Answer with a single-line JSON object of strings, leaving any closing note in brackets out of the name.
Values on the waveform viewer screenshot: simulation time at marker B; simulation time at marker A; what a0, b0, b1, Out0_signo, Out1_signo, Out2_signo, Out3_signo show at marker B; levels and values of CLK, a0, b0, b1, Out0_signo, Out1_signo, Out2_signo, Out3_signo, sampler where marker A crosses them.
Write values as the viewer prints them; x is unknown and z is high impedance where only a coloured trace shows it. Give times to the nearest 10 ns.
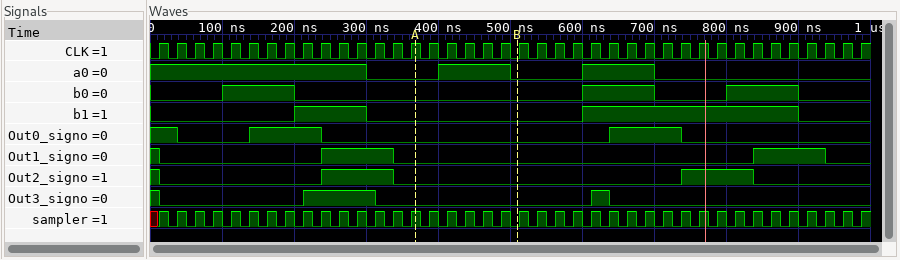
{"simulation time at marker B": "510 ns", "simulation time at marker A": "370 ns", "what a0, b0, b1, Out0_signo, Out1_signo, Out2_signo, Out3_signo show at marker B": "a0=0, b0=0, b1=0, Out0_signo=0, Out1_signo=0, Out2_signo=0, Out3_signo=0", "levels and values of CLK, a0, b0, b1, Out0_signo, Out1_signo, Out2_signo, Out3_signo, sampler where marker A crosses them": "CLK=1, a0=0, b0=0, b1=0, Out0_signo=0, Out1_signo=0, Out2_signo=0, Out3_signo=0, sampler=1"}
